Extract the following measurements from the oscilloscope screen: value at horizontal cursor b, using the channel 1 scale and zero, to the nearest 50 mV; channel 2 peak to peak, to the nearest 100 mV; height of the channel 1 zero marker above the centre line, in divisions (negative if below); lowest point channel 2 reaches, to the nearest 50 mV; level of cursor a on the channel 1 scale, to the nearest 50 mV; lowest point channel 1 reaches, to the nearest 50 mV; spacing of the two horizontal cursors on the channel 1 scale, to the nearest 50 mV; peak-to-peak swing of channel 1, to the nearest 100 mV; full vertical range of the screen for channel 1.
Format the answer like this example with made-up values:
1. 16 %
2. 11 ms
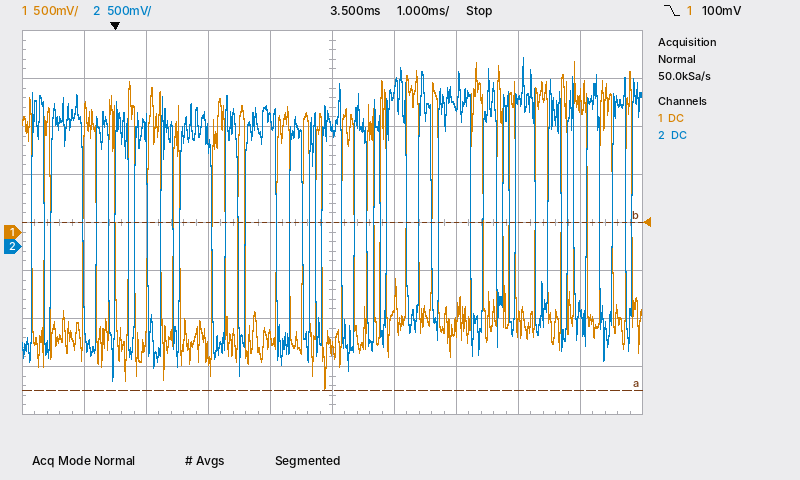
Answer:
1. 100 mV
2. 3.40 V
3. -0.2 div
4. -1.40 V
5. -1.65 V
6. -1.65 V
7. 1.75 V
8. 3.40 V
9. 4 V
